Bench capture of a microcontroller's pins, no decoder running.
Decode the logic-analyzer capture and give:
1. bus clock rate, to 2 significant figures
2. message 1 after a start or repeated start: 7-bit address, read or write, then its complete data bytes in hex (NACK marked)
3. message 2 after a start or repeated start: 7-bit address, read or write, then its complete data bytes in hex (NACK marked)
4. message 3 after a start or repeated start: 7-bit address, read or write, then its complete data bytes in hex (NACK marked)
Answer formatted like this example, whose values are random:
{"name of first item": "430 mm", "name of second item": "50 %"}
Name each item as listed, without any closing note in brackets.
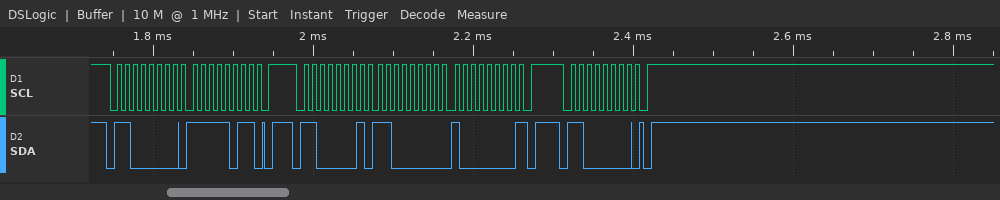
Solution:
{"bus clock rate, to 2 significant figures": "100 kHz", "message 1 after a start or repeated start: 7-bit address, read or write, then its complete data bytes in hex": "0x60 write: FB", "message 2 after a start or repeated start: 7-bit address, read or write, then its complete data bytes in hex": "0x60 read: C0 80 NACK", "message 3 after a start or repeated start: 7-bit address, read or write, then its complete data bytes in hex": "0x60 write"}
